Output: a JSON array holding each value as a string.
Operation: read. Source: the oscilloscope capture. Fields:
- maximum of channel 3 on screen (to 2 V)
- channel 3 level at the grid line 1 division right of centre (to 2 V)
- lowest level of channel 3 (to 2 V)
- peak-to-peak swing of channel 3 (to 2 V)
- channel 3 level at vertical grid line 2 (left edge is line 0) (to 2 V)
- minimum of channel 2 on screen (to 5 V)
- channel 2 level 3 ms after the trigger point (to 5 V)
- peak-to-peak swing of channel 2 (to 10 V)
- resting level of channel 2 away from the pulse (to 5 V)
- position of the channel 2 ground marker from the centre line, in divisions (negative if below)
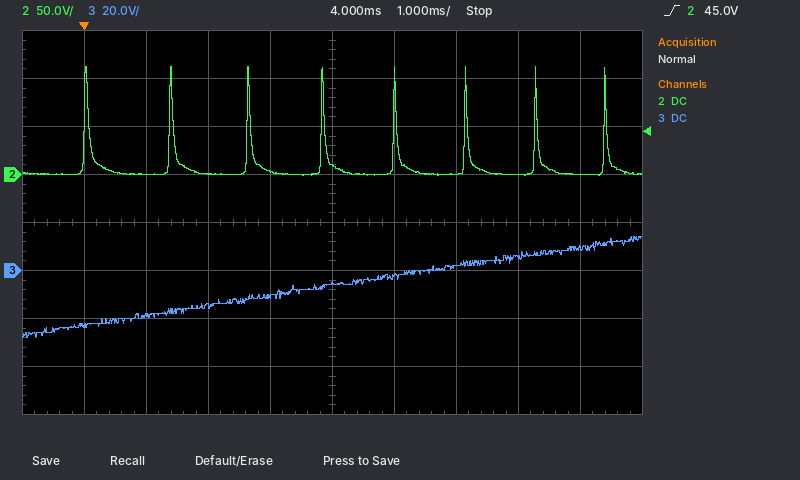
["14 V", "-2 V", "-28 V", "42 V", "-18 V", "0 V", "5 V", "110 V", "0 V", "+1.0 div"]
